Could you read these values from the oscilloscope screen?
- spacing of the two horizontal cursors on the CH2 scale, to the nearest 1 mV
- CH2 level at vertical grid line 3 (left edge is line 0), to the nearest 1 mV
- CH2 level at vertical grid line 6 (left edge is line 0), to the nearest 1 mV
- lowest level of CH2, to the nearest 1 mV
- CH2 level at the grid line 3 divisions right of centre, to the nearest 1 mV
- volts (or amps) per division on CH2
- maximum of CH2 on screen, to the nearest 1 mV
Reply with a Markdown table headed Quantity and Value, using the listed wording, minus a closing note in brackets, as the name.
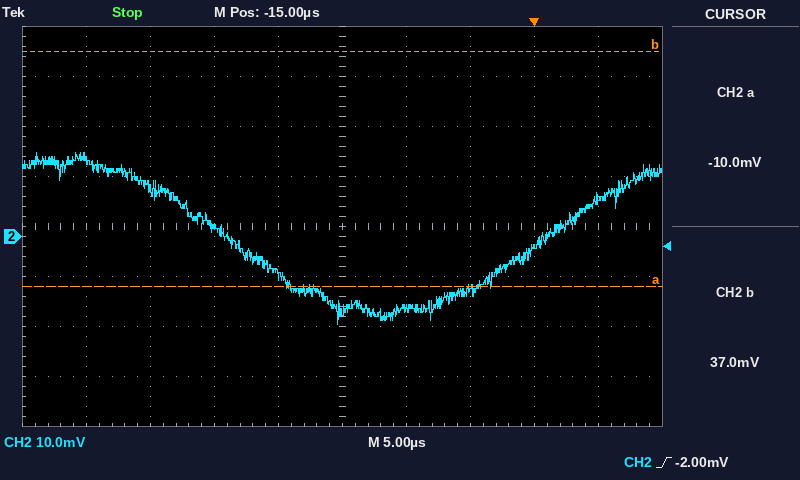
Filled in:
| Quantity | Value |
|---|---|
| spacing of the two horizontal cursors on the CH2 scale, to the nearest 1 mV | 47 mV |
| CH2 level at vertical grid line 3 (left edge is line 0), to the nearest 1 mV | 2 mV |
| CH2 level at vertical grid line 6 (left edge is line 0), to the nearest 1 mV | -14 mV |
| lowest level of CH2, to the nearest 1 mV | -18 mV |
| CH2 level at the grid line 3 divisions right of centre, to the nearest 1 mV | -2 mV |
| volts (or amps) per division on CH2 | 10 mV |
| maximum of CH2 on screen, to the nearest 1 mV | 17 mV |
